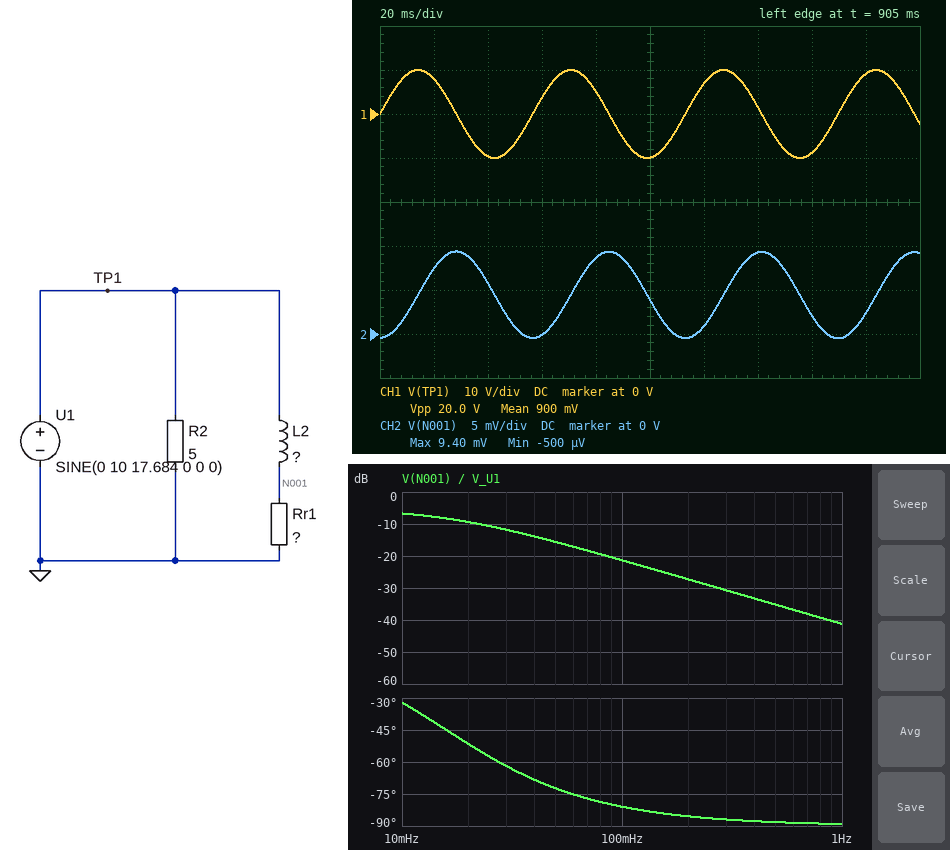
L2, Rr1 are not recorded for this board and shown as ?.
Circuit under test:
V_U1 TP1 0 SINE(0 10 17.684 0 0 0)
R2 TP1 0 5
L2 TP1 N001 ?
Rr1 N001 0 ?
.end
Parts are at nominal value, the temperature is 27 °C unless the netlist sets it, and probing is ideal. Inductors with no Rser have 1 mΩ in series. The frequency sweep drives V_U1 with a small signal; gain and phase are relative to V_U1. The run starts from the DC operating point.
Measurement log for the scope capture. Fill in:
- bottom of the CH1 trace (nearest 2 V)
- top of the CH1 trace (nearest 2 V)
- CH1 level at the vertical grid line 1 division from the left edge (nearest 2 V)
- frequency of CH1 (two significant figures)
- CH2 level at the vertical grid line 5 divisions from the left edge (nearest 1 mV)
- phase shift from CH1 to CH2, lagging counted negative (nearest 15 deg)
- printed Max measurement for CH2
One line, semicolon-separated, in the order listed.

-10 V; 10 V; 8 V; 18 Hz; 4 mV; -90 deg; 9.40 mV
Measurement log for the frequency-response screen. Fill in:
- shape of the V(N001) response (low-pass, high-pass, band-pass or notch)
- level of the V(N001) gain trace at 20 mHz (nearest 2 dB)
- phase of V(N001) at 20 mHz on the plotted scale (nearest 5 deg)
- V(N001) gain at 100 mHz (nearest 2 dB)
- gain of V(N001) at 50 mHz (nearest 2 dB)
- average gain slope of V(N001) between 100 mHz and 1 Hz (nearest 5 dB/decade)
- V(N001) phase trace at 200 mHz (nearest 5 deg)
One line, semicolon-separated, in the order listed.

low-pass; -10 dB; -50 deg; -22 dB; -16 dB; -20 dB/decade; -85 deg
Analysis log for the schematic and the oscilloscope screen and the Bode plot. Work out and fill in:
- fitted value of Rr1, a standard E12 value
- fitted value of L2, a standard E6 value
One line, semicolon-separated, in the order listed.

1.2 mΩ; 22 mH
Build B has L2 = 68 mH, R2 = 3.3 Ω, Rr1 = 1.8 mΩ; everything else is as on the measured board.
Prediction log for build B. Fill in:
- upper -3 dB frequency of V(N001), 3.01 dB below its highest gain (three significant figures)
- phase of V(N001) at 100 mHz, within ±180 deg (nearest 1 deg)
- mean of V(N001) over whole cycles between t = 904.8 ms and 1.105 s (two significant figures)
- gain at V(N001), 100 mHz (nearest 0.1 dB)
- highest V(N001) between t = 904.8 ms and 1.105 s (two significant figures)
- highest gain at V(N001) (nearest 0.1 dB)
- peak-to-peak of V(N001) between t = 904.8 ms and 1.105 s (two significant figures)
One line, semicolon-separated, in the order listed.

6.55 mHz; -86 deg; 2.3 mV; -27.5 dB; 4.7 mV; -3.8 dB; 4.8 mV
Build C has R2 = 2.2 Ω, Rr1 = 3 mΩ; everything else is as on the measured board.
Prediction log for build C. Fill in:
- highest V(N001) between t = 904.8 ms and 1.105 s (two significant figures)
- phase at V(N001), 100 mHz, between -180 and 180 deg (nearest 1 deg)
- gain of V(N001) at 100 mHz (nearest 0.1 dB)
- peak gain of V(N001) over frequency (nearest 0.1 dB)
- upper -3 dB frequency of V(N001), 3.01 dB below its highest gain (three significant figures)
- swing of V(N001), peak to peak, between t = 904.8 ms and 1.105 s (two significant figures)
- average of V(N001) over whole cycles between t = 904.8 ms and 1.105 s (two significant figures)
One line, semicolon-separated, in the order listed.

23 mV; -74 deg; -13.6 dB; -2.5 dB; 28.9 mHz; 25 mV; 10 mV
